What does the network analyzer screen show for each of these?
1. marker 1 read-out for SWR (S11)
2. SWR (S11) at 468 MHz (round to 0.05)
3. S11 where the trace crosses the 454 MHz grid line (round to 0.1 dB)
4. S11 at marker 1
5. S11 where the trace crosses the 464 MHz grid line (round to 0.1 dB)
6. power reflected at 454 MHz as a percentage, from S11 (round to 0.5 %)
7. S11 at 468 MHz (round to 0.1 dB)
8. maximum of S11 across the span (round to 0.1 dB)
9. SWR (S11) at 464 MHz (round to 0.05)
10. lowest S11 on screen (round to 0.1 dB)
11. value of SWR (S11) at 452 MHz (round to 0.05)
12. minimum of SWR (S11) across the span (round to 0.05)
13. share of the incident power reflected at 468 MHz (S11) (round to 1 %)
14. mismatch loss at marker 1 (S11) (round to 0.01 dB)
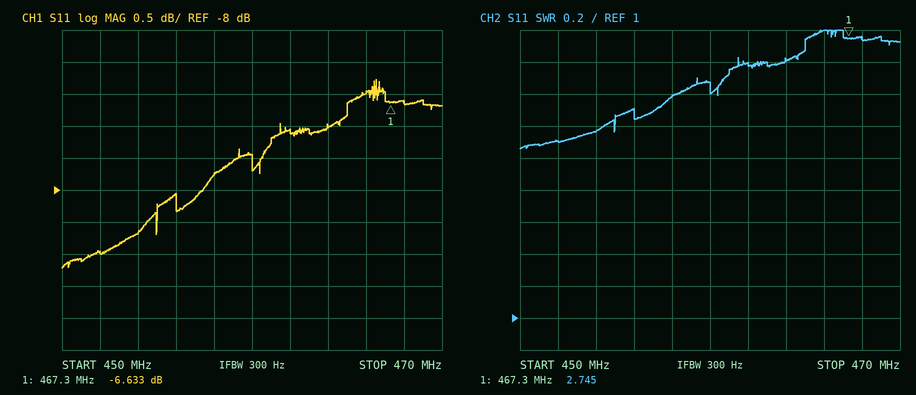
2.745
2.75
-8.7 dB
-6.633 dB
-7.0 dB
13.5 %
-6.6 dB
-6.3 dB
2.60
-9.2 dB
2.10
2.05
22 %
1.06 dB
